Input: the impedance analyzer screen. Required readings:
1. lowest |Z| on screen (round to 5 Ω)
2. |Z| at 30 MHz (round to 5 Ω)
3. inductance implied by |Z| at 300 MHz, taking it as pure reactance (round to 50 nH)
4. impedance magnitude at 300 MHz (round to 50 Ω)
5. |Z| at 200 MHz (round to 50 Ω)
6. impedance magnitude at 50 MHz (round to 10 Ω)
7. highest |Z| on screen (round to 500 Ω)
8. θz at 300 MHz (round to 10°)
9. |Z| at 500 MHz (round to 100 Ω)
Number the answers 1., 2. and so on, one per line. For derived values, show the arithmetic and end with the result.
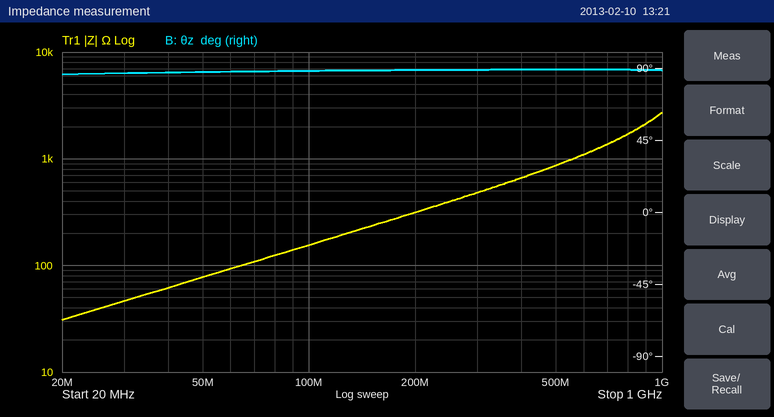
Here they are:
1. 30 Ω
2. 45 Ω
3. L = 500 Ω/(2π × 300 MHz) ≈ 265 nH, so 250 nH to the nearest 50 nH
4. 500 Ω
5. 300 Ω
6. 80 Ω
7. 2.5 kΩ
8. 90°
9. 900 Ω
